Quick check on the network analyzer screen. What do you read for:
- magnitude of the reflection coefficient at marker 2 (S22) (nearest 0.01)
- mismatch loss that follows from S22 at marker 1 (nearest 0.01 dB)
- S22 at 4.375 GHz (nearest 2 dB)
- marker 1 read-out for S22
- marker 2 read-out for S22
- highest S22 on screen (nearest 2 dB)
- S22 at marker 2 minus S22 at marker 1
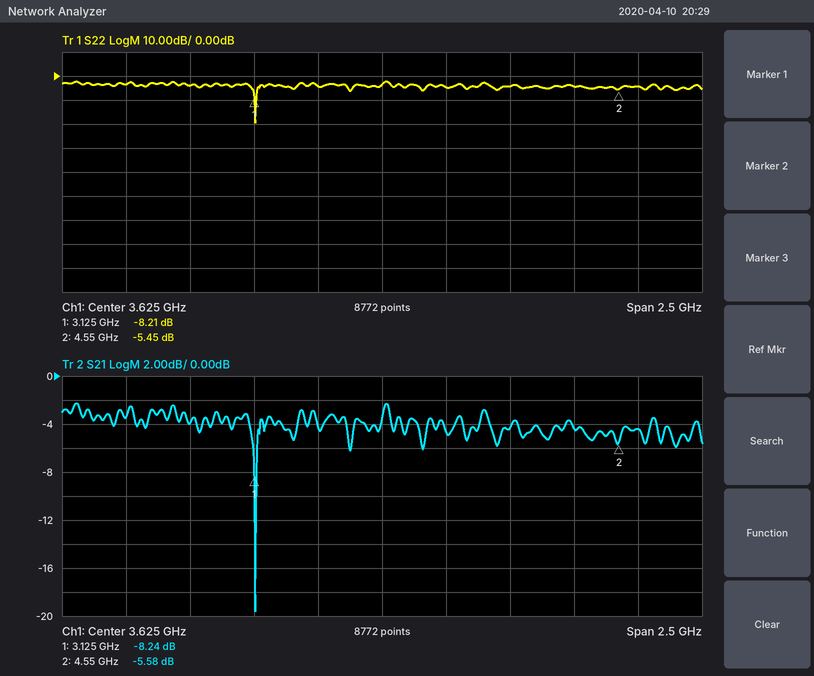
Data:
0.53
0.71 dB
-4 dB
-8.21 dB
-5.45 dB
-2 dB
2.76 dB
